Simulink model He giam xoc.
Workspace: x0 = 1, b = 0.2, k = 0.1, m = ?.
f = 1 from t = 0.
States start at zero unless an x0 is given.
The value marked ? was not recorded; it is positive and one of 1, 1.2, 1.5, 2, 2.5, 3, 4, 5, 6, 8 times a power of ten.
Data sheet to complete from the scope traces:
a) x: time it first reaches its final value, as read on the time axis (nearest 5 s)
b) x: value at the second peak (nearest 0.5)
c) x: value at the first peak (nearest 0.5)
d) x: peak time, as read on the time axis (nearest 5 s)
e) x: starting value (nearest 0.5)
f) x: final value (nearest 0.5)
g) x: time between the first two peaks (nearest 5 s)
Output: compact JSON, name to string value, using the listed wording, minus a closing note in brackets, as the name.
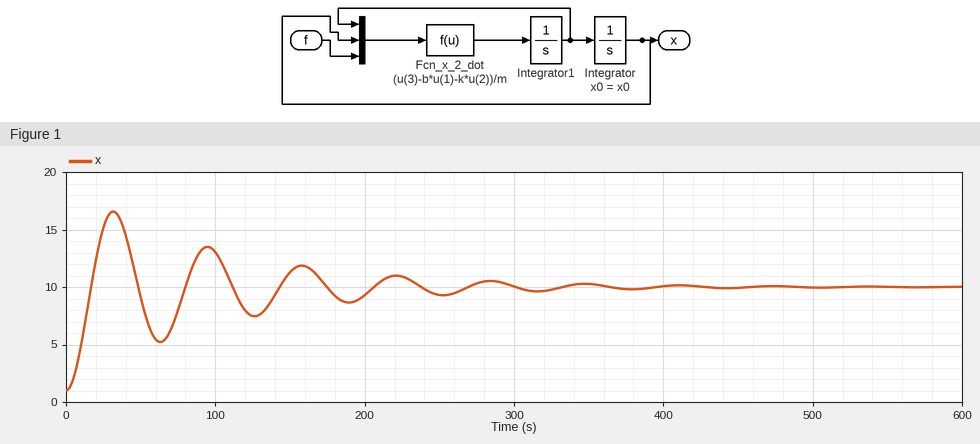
{"x: time it first reaches its final value, as read on the time axis": "15 s", "x: value at the second peak": "13.5", "x: value at the first peak": "16.5", "x: peak time, as read on the time axis": "30 s", "x: starting value": "1.0", "x: final value": "10.0", "x: time between the first two peaks": "65 s"}
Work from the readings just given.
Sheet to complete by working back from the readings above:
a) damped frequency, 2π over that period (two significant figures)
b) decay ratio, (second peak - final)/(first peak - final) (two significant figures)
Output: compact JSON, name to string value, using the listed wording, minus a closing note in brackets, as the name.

{"damped frequency, 2π over that period": "0.097 rad/s", "decay ratio, (second peak - final)/(first peak - final)": "0.54"}
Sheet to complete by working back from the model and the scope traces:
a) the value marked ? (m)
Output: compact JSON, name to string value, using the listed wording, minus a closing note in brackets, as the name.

{"the value marked ?": "10"}
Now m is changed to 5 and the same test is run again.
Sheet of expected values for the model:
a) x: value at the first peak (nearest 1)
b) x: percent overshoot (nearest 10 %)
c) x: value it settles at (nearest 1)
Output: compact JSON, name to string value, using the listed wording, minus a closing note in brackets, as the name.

{"x: value at the first peak": "16", "x: percent overshoot": "60 %", "x: value it settles at": "10"}
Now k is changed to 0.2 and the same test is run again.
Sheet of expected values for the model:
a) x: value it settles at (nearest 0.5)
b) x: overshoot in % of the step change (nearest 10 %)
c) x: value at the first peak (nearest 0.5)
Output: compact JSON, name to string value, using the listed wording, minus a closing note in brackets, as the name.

{"x: value it settles at": "5.0", "x: overshoot in % of the step change": "80 %", "x: value at the first peak": "8.0"}
